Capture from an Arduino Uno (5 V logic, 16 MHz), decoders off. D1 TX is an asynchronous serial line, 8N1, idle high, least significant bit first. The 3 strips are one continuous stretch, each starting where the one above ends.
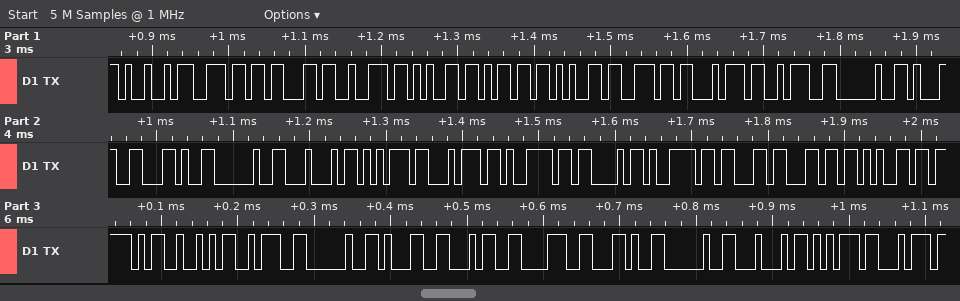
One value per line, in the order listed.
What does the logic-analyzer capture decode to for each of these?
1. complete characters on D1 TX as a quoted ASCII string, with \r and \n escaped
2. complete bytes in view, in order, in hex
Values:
"Increment: 1, DutyCycle_R: 148, Dut"
0x49 0x6E 0x63 0x72 0x65 0x6D 0x65 0x6E 0x74 0x3A 0x20 0x31 0x2C 0x20 0x44 0x75 0x74 0x79 0x43 0x79 0x63 0x6C 0x65 0x5F 0x52 0x3A 0x20 0x31 0x34 0x38 0x2C 0x20 0x44 0x75 0x74
